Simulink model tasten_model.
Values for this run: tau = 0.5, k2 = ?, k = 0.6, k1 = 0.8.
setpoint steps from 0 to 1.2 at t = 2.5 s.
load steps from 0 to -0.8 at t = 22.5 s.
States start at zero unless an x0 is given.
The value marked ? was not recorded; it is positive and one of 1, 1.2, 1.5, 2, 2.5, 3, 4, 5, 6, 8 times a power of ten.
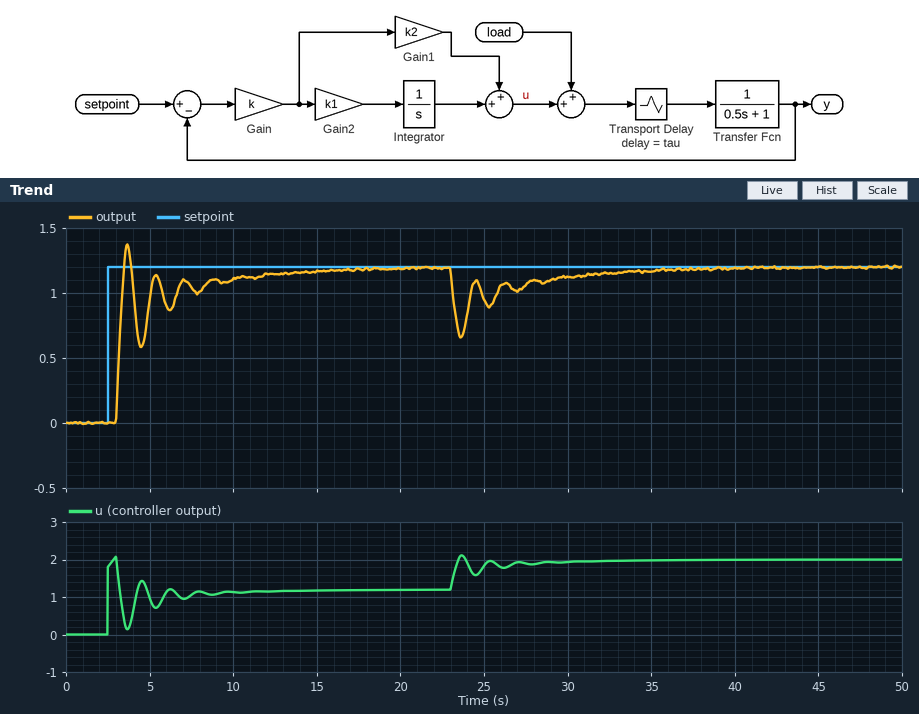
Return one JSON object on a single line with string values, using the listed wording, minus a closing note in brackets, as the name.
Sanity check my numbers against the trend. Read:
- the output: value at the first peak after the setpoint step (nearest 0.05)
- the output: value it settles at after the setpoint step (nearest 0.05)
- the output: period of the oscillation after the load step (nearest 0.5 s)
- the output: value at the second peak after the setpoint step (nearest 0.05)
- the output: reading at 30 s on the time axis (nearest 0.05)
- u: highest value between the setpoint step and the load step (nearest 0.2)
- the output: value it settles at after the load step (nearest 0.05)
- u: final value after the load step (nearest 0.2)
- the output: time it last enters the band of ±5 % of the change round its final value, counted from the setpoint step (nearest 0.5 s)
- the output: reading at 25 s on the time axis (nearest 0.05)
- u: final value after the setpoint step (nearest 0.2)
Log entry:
{"the output: value at the first peak after the setpoint step": "1.35", "the output: value it settles at after the setpoint step": "1.20", "the output: period of the oscillation after the load step": "1.5 s", "the output: value at the second peak after the setpoint step": "1.15", "the output: reading at 30 s on the time axis": "1.10", "u: highest value between the setpoint step and the load step": "2.0", "the output: value it settles at after the load step": "1.20", "u: final value after the load step": "2.0", "the output: time it last enters the band of ±5 % of the change round its final value, counted from the setpoint step": "9.5 s", "the output: reading at 25 s on the time axis": "0.95", "u: final value after the setpoint step": "1.2"}
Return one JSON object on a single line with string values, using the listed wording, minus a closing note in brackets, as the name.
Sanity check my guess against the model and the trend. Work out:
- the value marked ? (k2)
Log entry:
{"the value marked ?": "2.5"}
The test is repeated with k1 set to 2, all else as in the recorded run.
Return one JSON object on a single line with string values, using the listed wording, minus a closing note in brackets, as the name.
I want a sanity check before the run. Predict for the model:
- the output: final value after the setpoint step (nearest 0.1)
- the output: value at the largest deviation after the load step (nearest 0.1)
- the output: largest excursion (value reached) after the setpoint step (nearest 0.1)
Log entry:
{"the output: final value after the setpoint step": "1.2", "the output: value at the largest deviation after the load step": "0.7", "the output: largest excursion (value reached) after the setpoint step": "1.6"}
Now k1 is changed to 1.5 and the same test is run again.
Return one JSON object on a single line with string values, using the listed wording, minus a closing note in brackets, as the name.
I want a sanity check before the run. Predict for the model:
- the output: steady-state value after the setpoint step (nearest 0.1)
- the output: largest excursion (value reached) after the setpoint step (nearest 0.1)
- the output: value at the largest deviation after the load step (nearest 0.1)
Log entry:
{"the output: steady-state value after the setpoint step": "1.2", "the output: largest excursion (value reached) after the setpoint step": "1.5", "the output: value at the largest deviation after the load step": "0.7"}
